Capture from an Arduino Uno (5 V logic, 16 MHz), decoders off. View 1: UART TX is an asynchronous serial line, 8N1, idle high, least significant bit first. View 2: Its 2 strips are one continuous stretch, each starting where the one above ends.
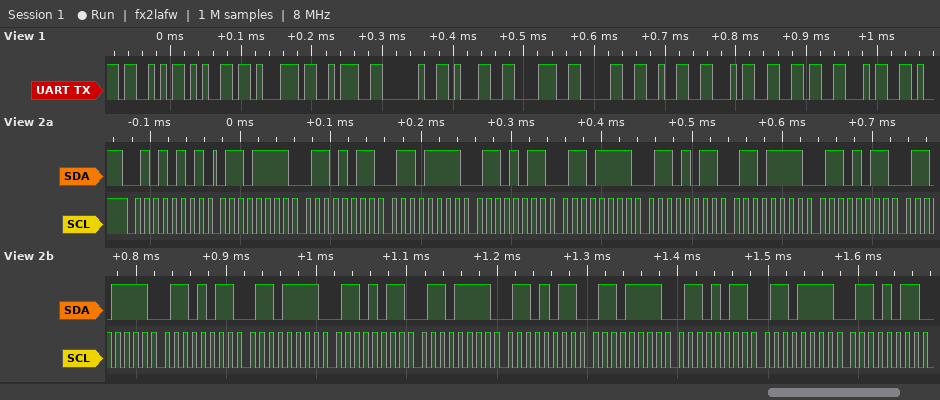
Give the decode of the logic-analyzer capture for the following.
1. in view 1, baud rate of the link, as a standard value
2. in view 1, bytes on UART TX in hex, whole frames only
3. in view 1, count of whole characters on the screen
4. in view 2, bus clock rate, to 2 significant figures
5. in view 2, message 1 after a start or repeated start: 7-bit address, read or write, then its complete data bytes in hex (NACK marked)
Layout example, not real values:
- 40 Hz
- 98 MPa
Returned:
- 115200 baud
- 53 65 71 3A 20 31 38 30 32 34 36 34
- 12
- 100 kHz
- 0x2A read: 6F 6B 6F 6B 6F 6B 6F 6B 6F 6B 6F 6B 6F 6B 6F 6B 6F 6B
